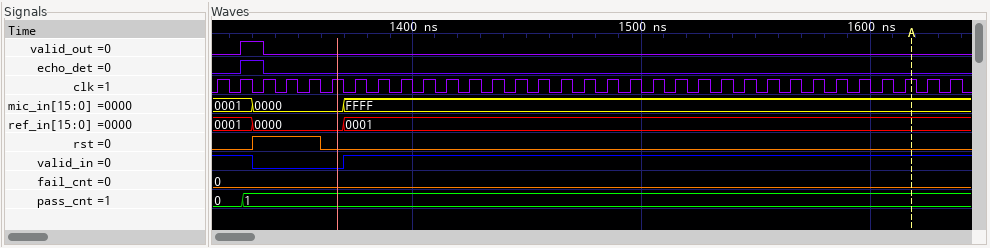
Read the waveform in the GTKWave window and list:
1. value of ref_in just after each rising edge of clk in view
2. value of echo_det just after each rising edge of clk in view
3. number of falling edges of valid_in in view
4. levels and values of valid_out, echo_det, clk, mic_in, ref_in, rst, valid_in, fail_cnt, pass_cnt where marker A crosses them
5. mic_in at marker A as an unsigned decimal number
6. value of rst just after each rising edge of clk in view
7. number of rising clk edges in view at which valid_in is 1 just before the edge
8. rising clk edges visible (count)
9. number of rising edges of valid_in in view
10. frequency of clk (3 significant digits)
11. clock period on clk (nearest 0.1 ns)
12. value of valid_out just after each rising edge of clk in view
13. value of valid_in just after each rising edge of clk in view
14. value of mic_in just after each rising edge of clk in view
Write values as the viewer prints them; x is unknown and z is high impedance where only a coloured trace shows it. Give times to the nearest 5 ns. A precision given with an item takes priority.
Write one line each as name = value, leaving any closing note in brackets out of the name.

value of ref_in just after each rising edge of clk in view = 0001, 0001, 0000, 0000, 0000, 0000, 0001, 0001, 0001, 0001, 0001, 0001, 0001, 0001, 0001, 0001, 0001, 0001, 0001, 0001, 0001, 0001, 0001, 0001, 0001, 0001, 0001, 0001, 0001, 0001, 0001, 0001, 0001
value of echo_det just after each rising edge of clk in view = 0 1 0 0 0 0 0 0 0 0 0 0 0 0 0 0 0 0 0 0 0 0 0 0 0 0 0 0 0 0 0 0 0
number of falling edges of valid_in in view = 1
levels and values of valid_out, echo_det, clk, mic_in, ref_in, rst, valid_in, fail_cnt, pass_cnt where marker A crosses them = valid_out=0, echo_det=0, clk=1, mic_in=FFFF, ref_in=0001, rst=0, valid_in=1, fail_cnt=0, pass_cnt=1
mic_in at marker A as an unsigned decimal number = 65535
value of rst just after each rising edge of clk in view = 0 0 1 1 1 0 0 0 0 0 0 0 0 0 0 0 0 0 0 0 0 0 0 0 0 0 0 0 0 0 0 0 0
number of rising clk edges in view at which valid_in is 1 just before the edge = 29
rising clk edges visible = 33
number of rising edges of valid_in in view = 1
frequency of clk = 100 MHz
clock period on clk = 10 ns
value of valid_out just after each rising edge of clk in view = 0 1 0 0 0 0 0 0 0 0 0 0 0 0 0 0 0 0 0 0 0 0 0 0 0 0 0 0 0 0 0 0 0
value of valid_in just after each rising edge of clk in view = 1 1 0 0 0 0 1 1 1 1 1 1 1 1 1 1 1 1 1 1 1 1 1 1 1 1 1 1 1 1 1 1 1
value of mic_in just after each rising edge of clk in view = 0001, 0001, 0000, 0000, 0000, 0000, FFFF, FFFF, FFFF, FFFF, FFFF, FFFF, FFFF, FFFF, FFFF, FFFF, FFFF, FFFF, FFFF, FFFF, FFFF, FFFF, FFFF, FFFF, FFFF, FFFF, FFFF, FFFF, FFFF, FFFF, FFFF, FFFF, FFFF
